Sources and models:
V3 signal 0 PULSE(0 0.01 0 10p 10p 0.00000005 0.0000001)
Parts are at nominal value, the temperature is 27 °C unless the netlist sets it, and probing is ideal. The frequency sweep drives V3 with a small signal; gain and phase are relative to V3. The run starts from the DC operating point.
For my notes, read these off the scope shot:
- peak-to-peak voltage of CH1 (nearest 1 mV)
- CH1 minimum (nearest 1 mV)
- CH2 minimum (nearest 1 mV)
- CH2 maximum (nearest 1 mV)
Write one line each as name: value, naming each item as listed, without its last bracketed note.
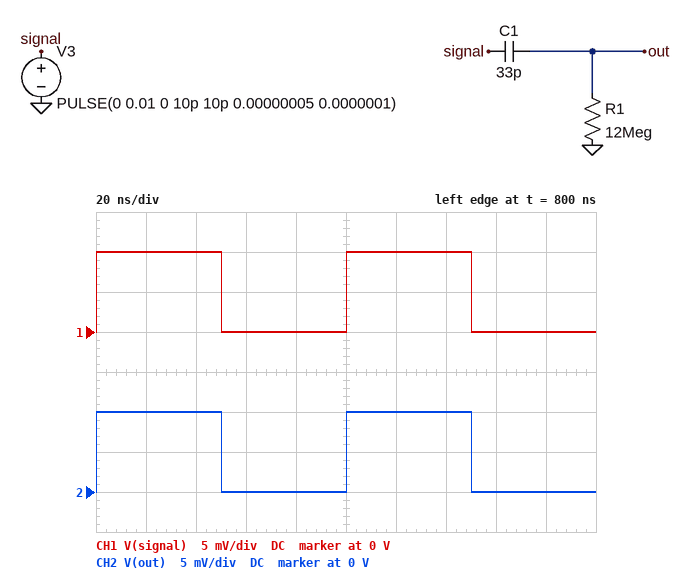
peak-to-peak voltage of CH1: 10 mV
CH1 minimum: 0 V
CH2 minimum: 0 V
CH2 maximum: 10 mV
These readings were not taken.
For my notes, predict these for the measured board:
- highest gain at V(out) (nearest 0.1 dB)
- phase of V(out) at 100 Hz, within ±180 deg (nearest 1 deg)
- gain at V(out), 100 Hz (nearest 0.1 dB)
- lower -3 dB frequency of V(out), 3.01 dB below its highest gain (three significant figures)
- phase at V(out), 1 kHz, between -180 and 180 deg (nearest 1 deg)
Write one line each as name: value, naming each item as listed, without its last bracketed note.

highest gain at V(out): 0 dB
phase of V(out) at 100 Hz, within ±180 deg: 76 deg
gain at V(out), 100 Hz: -12.3 dB
lower -3 dB frequency of V(out), 3.01 dB below its highest gain: 402 Hz
phase at V(out), 1 kHz, between -180 and 180 deg: 22 deg
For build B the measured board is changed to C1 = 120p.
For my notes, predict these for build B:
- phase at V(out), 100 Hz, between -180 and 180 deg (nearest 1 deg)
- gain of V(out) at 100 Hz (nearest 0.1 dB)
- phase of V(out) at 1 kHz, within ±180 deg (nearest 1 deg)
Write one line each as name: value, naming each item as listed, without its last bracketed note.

phase at V(out), 100 Hz, between -180 and 180 deg: 48 deg
gain of V(out) at 100 Hz: -3.5 dB
phase of V(out) at 1 kHz, within ±180 deg: 6 deg
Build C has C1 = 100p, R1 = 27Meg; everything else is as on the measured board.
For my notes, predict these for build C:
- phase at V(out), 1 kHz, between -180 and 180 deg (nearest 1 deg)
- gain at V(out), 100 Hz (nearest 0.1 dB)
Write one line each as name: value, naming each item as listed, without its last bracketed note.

phase at V(out), 1 kHz, between -180 and 180 deg: 3 deg
gain at V(out), 100 Hz: -1.3 dB
